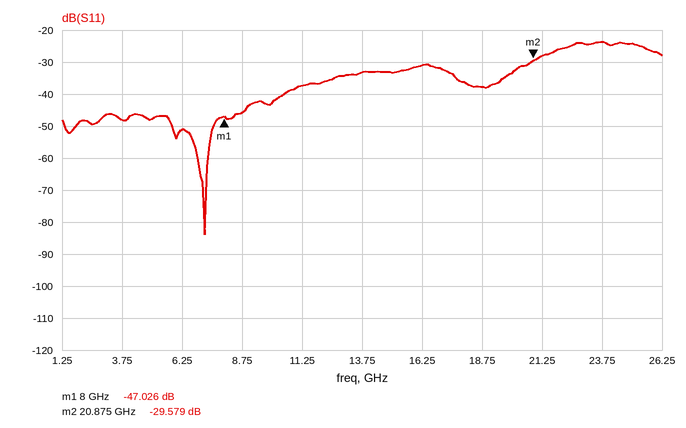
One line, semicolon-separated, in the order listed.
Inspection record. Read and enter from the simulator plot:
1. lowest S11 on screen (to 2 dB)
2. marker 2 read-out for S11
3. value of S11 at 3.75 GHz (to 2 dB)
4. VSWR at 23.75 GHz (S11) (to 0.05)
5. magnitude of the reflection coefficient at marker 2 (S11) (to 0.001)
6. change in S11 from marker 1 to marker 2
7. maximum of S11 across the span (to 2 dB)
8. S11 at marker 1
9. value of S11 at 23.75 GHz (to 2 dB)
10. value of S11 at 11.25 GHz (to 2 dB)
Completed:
-84 dB; -29.579 dB; -48 dB; 1.15; 0.033; 17.447 dB; -24 dB; -47.026 dB; -24 dB; -38 dB
